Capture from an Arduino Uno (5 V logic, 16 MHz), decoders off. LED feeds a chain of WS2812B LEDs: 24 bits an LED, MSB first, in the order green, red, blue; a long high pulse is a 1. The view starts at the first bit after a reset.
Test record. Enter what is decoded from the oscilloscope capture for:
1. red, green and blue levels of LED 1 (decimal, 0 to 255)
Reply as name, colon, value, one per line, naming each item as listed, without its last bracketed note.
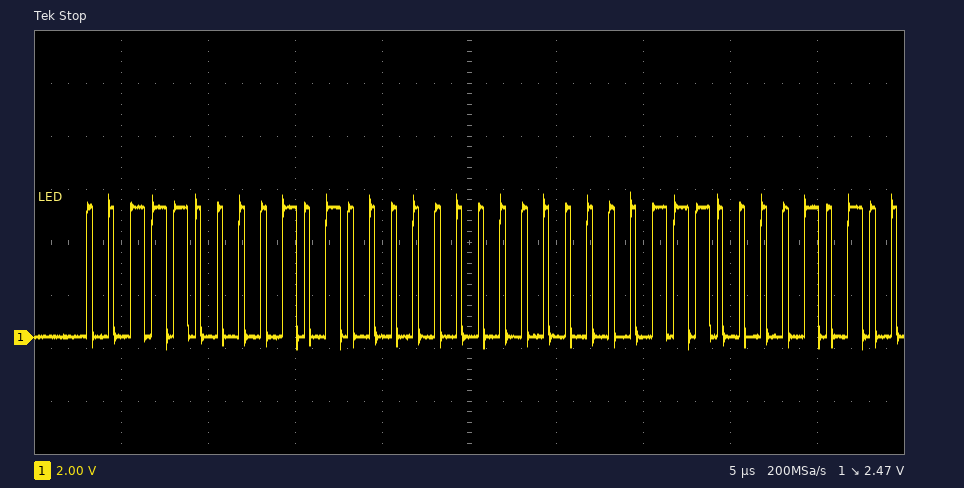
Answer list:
red, green and blue levels of LED 1: 80, 56, 0
